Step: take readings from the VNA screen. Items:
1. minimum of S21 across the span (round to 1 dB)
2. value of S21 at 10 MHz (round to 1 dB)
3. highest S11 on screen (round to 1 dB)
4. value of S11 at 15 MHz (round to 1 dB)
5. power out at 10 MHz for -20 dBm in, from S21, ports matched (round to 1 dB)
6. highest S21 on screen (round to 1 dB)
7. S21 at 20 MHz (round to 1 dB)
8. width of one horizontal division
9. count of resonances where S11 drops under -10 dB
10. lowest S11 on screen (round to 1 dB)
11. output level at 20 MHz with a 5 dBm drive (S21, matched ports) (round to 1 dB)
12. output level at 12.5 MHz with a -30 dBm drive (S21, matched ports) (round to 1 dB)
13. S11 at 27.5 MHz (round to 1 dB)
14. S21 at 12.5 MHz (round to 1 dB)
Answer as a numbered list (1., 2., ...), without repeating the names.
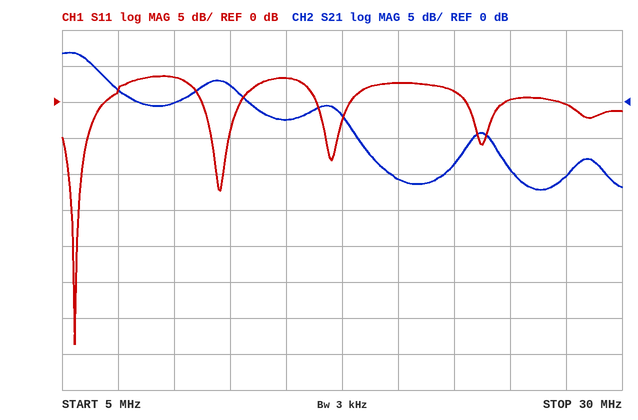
1. -12 dB
2. 0 dB
3. 4 dB
4. 3 dB
5. -20 dBm
6. 7 dB
7. -11 dB
8. 2.5 MHz
9. 2
10. -34 dB
11. -6 dBm
12. -28 dBm
13. 0 dB
14. 2 dB
